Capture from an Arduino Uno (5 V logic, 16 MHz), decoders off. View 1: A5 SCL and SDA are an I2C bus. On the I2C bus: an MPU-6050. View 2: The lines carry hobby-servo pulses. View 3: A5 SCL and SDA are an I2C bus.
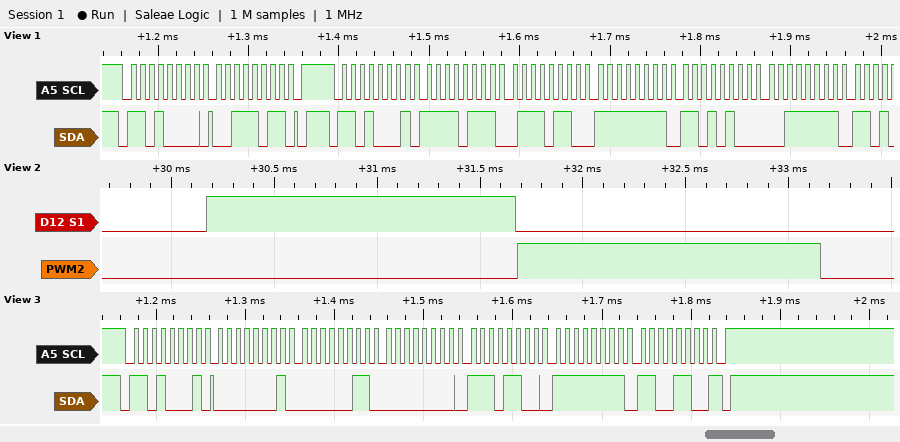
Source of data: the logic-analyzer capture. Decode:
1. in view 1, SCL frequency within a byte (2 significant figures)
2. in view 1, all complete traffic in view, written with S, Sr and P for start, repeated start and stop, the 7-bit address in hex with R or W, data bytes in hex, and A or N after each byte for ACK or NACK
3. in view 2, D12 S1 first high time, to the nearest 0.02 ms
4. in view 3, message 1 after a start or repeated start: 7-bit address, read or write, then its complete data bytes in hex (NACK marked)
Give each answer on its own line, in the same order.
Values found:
100 kHz
S 68W A 3B A P S 68R A F7 A 76 A FF A D4 A 3F A
1.50 ms
0x68 read: 01 03 00 EC FF CC NACK
